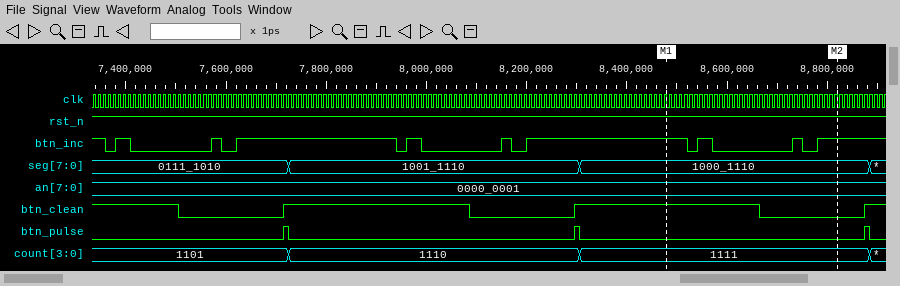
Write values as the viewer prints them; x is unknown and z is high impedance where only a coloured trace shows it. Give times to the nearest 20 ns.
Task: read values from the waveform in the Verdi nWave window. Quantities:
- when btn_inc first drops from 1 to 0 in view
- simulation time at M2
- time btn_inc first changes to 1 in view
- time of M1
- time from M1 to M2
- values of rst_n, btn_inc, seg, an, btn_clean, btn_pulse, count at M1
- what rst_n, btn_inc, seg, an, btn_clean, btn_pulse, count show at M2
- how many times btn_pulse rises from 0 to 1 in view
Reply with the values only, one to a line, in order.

7360 ns
8820 ns
7380 ns
8480 ns
340 ns
rst_n=1, btn_inc=1, seg=1000_1110, an=0000_0001, btn_clean=1, btn_pulse=0, count=1111
rst_n=1, btn_inc=1, seg=1000_1110, an=0000_0001, btn_clean=0, btn_pulse=0, count=1111
3
